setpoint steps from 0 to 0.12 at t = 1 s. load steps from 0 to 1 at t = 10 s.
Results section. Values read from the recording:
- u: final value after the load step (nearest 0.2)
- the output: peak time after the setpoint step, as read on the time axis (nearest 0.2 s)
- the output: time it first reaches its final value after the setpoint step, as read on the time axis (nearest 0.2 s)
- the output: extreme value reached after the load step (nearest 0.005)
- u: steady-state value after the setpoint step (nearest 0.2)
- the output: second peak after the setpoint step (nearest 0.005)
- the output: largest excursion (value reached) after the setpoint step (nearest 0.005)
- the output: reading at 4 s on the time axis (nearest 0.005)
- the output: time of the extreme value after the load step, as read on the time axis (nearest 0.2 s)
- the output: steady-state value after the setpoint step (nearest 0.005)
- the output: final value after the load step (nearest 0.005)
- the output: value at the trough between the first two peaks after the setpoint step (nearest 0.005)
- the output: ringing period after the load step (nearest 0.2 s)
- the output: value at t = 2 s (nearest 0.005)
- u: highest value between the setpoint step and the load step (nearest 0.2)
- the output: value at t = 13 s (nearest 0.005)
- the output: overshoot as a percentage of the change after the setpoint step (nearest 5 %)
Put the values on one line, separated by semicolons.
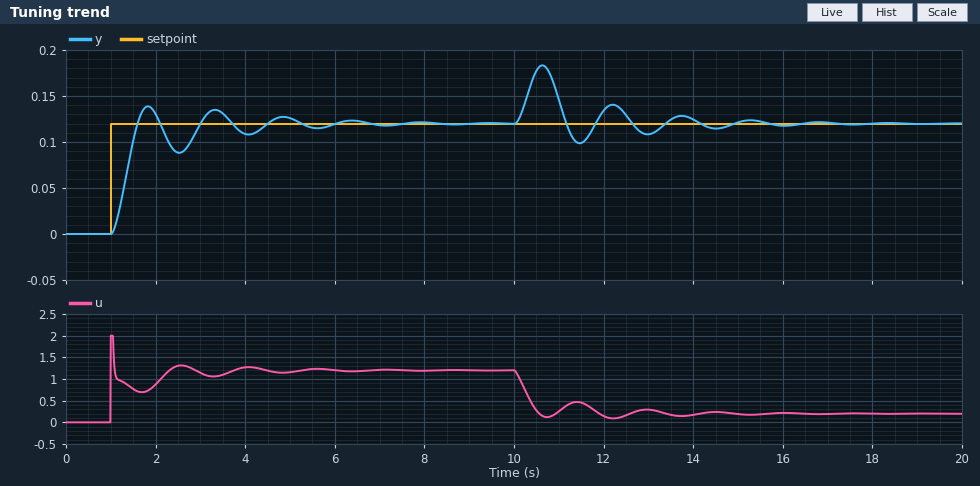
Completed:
0.2; 1.8 s; 1.6 s; 0.185; 1.2; 0.135; 0.140; 0.110; 10.6 s; 0.120; 0.120; 0.090; 1.6 s; 0.130; 2.0; 0.110; 15 %
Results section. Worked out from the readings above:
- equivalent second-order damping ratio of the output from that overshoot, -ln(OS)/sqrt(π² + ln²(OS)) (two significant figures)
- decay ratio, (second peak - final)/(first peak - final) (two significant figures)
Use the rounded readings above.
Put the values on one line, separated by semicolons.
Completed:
0.52; 0.75
